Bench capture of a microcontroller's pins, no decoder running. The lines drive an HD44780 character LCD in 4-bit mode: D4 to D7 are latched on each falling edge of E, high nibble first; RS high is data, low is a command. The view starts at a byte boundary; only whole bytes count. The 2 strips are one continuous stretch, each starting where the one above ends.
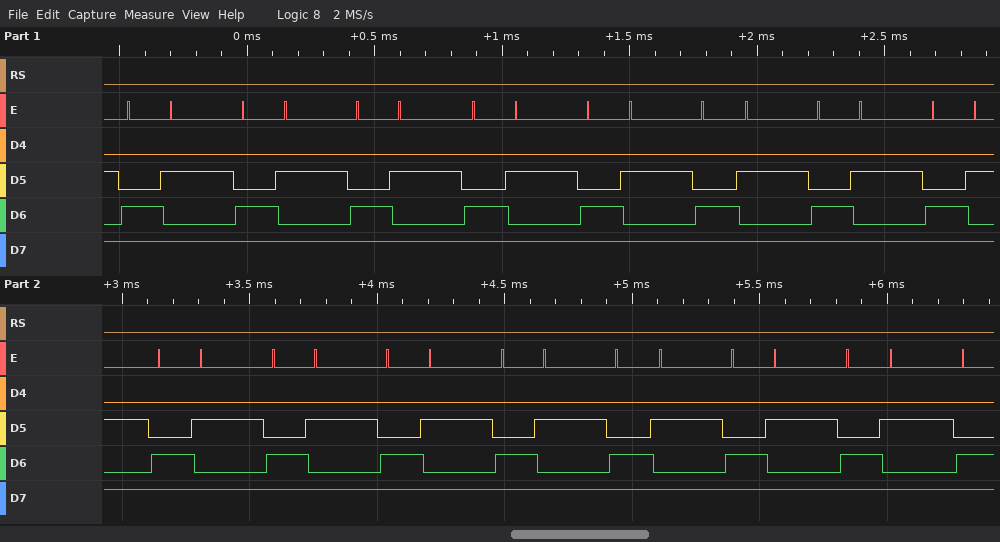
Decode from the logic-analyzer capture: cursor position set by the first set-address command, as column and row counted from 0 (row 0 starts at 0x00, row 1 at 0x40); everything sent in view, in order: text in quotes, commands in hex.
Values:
column 10, row 1
0xCA 0xCA 0xCA 0xCA 0xCA 0xCA 0xCA 0xCA 0xCA 0xCA 0xCA 0xCA 0xCA 0xCA 0xCA
